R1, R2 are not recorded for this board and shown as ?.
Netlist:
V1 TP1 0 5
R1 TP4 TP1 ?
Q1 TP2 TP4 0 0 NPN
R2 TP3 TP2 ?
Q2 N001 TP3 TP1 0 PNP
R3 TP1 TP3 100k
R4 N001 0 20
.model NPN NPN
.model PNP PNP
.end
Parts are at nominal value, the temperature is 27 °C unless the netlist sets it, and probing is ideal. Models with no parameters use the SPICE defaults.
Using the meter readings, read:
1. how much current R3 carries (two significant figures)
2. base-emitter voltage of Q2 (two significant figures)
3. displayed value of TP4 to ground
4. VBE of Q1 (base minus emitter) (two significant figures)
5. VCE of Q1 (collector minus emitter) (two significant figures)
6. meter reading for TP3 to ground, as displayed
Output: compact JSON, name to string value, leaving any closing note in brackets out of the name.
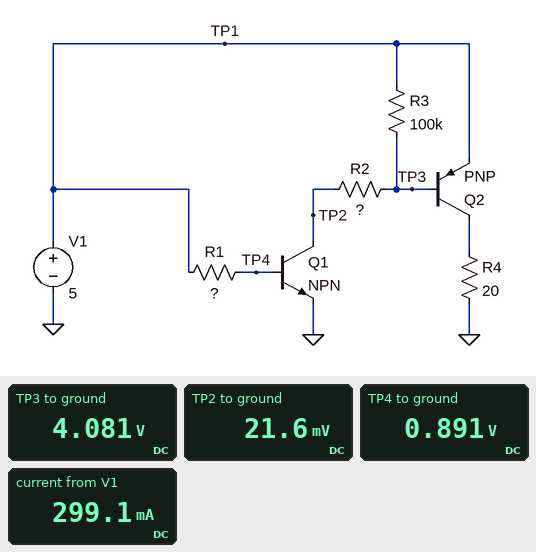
{"how much current R3 carries": "9.2 µA", "base-emitter voltage of Q2": "-920 mV", "displayed value of TP4 to ground": "0.891 V", "VBE of Q1 (base minus emitter)": "890 mV", "VCE of Q1 (collector minus emitter)": "22 mV", "meter reading for TP3 to ground, as displayed": "4.081 V"}
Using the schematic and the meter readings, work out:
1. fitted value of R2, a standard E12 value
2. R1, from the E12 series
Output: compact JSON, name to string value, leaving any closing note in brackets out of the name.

{"fitted value of R2, a standard E12 value": "330 Ω", "R1, from the E12 series": "100 Ω"}
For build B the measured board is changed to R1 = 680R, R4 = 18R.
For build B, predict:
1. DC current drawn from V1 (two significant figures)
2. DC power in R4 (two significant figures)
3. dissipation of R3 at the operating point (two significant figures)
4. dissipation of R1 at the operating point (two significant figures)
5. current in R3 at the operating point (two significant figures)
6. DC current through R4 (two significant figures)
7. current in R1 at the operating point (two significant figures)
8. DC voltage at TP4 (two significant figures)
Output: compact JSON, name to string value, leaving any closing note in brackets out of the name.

{"DC current drawn from V1": "290 mA", "DC power in R4": "1.3 W", "dissipation of R3 at the operating point": "8.5 µW", "dissipation of R1 at the operating point": "25 mW", "current in R3 at the operating point": "9.2 µA", "DC current through R4": "270 mA", "current in R1 at the operating point": "6.1 mA", "DC voltage at TP4": "860 mV"}
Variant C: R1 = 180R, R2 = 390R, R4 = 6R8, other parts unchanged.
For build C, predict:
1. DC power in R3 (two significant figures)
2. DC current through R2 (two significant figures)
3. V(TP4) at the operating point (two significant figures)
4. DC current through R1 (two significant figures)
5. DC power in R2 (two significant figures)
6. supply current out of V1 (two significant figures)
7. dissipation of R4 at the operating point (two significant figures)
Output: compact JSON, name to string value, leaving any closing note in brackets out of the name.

{"DC power in R3": "8.9 µW", "DC current through R2": "10 mA", "V(TP4) at the operating point": "880 mV", "DC current through R1": "23 mA", "DC power in R2": "42 mW", "supply current out of V1": "750 mA", "dissipation of R4 at the operating point": "3.5 W"}
